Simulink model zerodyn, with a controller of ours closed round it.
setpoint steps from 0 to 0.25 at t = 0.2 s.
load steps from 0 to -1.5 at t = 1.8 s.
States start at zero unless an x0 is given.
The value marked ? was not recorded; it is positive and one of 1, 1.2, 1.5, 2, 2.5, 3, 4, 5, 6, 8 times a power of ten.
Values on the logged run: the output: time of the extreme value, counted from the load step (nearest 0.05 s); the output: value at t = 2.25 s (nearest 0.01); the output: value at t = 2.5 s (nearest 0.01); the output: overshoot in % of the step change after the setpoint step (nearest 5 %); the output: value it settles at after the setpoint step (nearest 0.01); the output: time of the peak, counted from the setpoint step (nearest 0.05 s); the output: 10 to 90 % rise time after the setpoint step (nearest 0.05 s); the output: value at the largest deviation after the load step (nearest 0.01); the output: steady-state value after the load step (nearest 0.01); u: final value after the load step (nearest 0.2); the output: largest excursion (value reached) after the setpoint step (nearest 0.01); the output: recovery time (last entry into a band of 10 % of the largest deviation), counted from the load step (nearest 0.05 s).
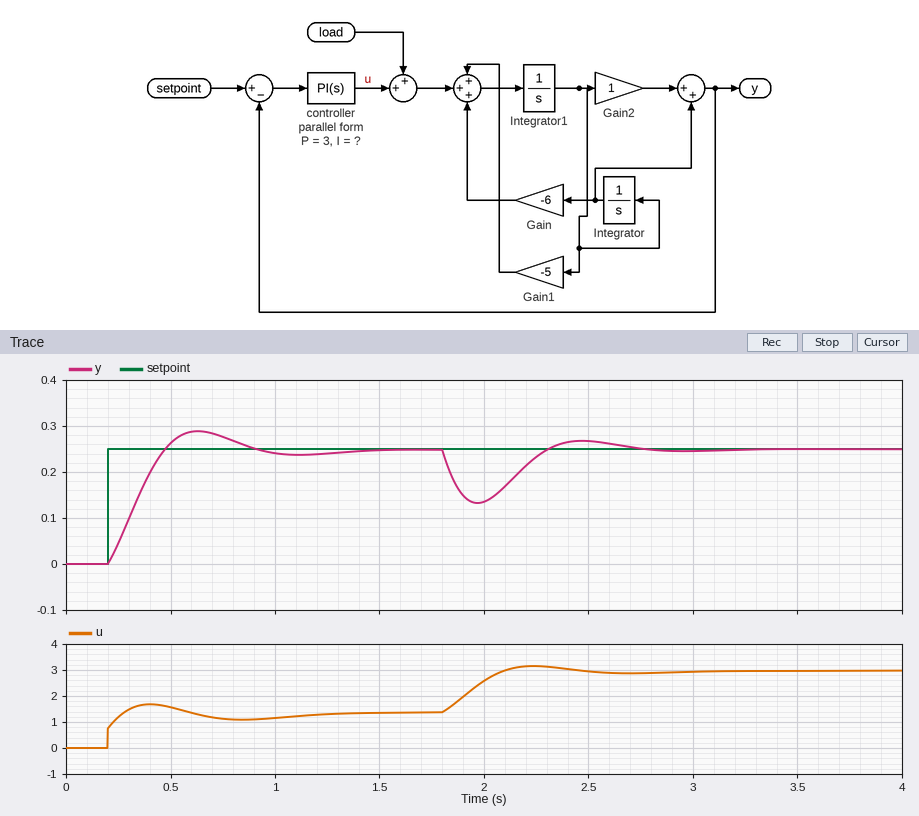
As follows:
0.15 s
0.23
0.27
15 %
0.25
0.45 s
0.20 s
0.13
0.25
3.0
0.29
0.80 s
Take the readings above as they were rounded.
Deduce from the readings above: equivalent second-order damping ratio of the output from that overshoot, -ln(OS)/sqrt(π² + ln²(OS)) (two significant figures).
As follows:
0.52
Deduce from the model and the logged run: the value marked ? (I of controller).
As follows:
50
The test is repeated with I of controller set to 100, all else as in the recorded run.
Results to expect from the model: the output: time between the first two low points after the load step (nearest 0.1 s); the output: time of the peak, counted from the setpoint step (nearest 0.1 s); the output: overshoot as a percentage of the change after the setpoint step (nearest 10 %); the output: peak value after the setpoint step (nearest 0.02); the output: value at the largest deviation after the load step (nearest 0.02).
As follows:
0.7 s
0.3 s
30 %
0.32
0.16
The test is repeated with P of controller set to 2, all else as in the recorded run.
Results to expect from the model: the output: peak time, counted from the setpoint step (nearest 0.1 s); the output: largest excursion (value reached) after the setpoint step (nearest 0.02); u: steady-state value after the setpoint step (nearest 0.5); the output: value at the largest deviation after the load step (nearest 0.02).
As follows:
0.4 s
0.30
1.5
0.12
